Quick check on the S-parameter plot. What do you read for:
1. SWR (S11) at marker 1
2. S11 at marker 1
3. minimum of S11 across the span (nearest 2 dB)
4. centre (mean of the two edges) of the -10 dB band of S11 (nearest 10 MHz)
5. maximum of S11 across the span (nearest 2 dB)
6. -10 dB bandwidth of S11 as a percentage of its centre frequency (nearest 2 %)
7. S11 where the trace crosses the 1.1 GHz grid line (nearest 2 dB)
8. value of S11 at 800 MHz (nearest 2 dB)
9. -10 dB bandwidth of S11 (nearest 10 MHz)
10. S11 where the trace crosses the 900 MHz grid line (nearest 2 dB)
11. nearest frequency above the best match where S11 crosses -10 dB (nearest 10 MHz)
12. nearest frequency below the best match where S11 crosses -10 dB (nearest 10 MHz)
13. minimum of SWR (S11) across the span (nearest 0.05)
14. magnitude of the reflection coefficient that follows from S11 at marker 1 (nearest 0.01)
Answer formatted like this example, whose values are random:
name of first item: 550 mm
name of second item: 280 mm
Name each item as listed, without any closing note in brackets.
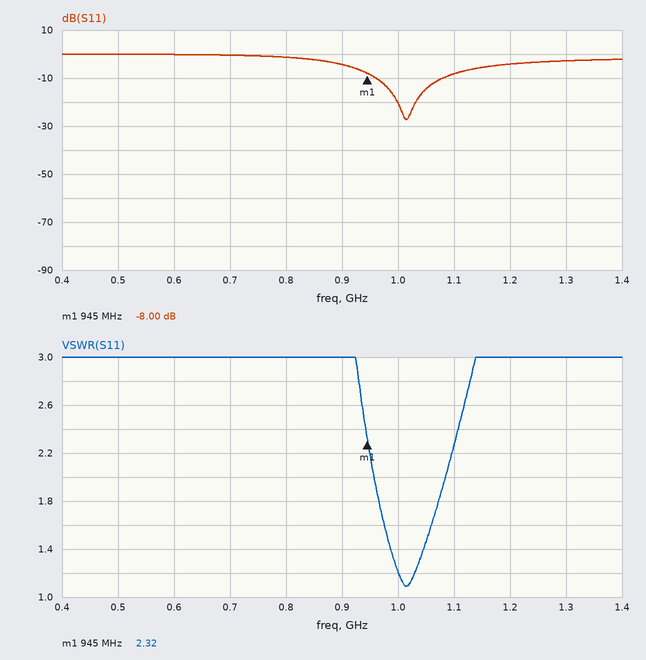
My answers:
SWR (S11) at marker 1: 2.32
S11 at marker 1: -8.00 dB
minimum of S11 across the span: -28 dB
centre (mean of the two edges) of the -10 dB band of S11: 1.02 GHz
maximum of S11 across the span: 0 dB
-10 dB bandwidth of S11 as a percentage of its centre frequency: 12 %
S11 where the trace crosses the 1.1 GHz grid line: -8 dB
value of S11 at 800 MHz: -2 dB
-10 dB bandwidth of S11: 120 MHz
S11 where the trace crosses the 900 MHz grid line: -4 dB
nearest frequency above the best match where S11 crosses -10 dB: 1.08 GHz
nearest frequency below the best match where S11 crosses -10 dB: 960 MHz
minimum of SWR (S11) across the span: 1.10
magnitude of the reflection coefficient that follows from S11 at marker 1: 0.40
